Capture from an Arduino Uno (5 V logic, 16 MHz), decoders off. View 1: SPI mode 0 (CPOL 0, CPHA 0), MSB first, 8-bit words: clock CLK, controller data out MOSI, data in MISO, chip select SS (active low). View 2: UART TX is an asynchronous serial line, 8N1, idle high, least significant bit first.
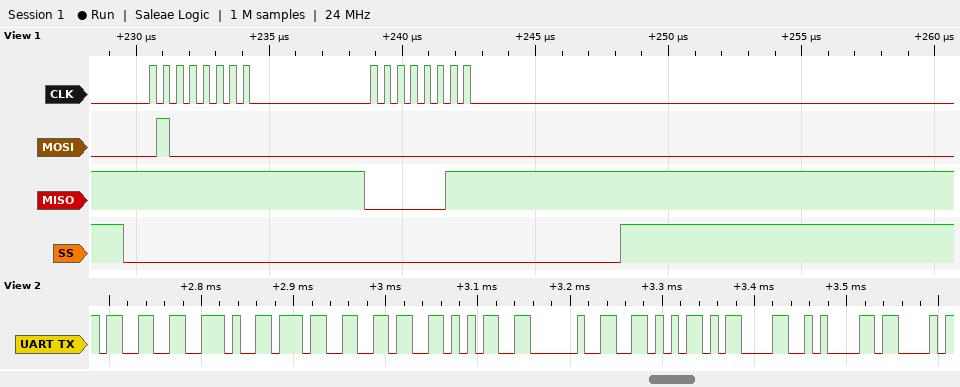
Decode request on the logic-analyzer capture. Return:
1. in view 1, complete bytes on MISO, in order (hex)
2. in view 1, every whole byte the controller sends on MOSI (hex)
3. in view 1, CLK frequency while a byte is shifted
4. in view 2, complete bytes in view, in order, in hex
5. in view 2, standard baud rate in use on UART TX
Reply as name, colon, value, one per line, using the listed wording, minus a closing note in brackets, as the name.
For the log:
in view 1, complete bytes on MISO, in order: FF 03
in view 1, every whole byte the controller sends on MOSI: 40 00
in view 1, CLK frequency while a byte is shifted: 2 MHz
in view 2, complete bytes in view, in order, in hex: 0x33 0x2E 0x37 0x36 0x35 0x20 0x56 0x0D 0x0A 0x43
in view 2, standard baud rate in use on UART TX: 115200 baud
